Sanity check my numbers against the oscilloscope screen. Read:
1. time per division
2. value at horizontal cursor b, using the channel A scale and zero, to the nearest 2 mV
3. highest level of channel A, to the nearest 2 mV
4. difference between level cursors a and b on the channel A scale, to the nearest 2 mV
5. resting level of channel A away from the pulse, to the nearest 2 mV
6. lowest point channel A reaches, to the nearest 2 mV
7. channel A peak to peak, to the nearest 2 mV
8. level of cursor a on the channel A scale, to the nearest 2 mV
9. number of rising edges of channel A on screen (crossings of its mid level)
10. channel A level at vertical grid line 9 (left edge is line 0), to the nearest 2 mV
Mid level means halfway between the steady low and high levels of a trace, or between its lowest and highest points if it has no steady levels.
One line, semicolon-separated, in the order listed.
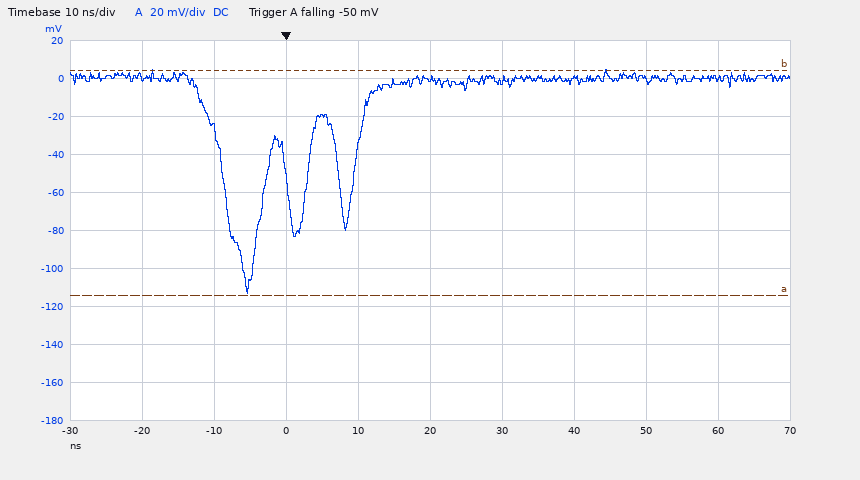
10 ns; 4 mV; 4 mV; 118 mV; 0 mV; -114 mV; 118 mV; -114 mV; 3; 0 mV
